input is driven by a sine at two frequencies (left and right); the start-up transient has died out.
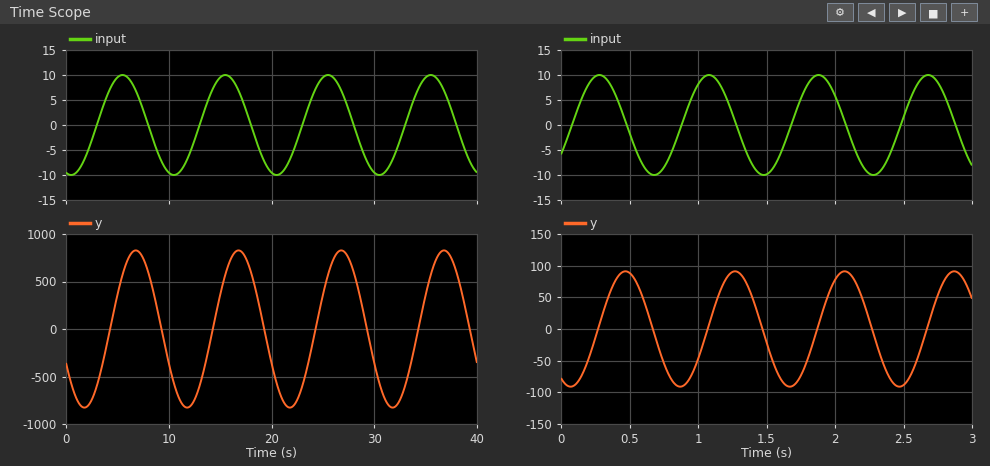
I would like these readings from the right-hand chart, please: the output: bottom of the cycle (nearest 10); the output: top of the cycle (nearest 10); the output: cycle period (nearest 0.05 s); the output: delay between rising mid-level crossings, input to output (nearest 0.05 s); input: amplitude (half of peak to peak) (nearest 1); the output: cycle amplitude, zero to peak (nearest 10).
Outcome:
-90
90
0.80 s
0.20 s
10
90
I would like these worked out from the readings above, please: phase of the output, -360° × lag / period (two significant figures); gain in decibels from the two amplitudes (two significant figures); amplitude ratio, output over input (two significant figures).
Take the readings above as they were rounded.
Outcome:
-90°
19 dB
9.0
